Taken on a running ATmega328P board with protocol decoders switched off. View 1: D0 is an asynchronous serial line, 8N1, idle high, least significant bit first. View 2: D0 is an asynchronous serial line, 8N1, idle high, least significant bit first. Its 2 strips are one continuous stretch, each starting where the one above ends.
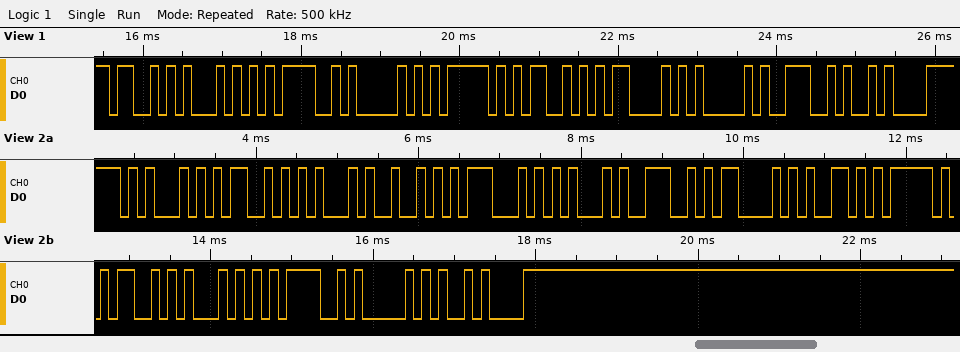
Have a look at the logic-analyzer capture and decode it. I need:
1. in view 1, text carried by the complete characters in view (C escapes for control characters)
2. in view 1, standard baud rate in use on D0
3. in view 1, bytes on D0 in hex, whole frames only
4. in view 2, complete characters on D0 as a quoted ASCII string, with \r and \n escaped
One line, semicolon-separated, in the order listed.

"STOP_SCAN\n"; 9600 baud; 0x53 0x54 0x4F 0x50 0x5F 0x53 0x43 0x41 0x4E 0x0A; "EMERGENCY_STOP\n"
